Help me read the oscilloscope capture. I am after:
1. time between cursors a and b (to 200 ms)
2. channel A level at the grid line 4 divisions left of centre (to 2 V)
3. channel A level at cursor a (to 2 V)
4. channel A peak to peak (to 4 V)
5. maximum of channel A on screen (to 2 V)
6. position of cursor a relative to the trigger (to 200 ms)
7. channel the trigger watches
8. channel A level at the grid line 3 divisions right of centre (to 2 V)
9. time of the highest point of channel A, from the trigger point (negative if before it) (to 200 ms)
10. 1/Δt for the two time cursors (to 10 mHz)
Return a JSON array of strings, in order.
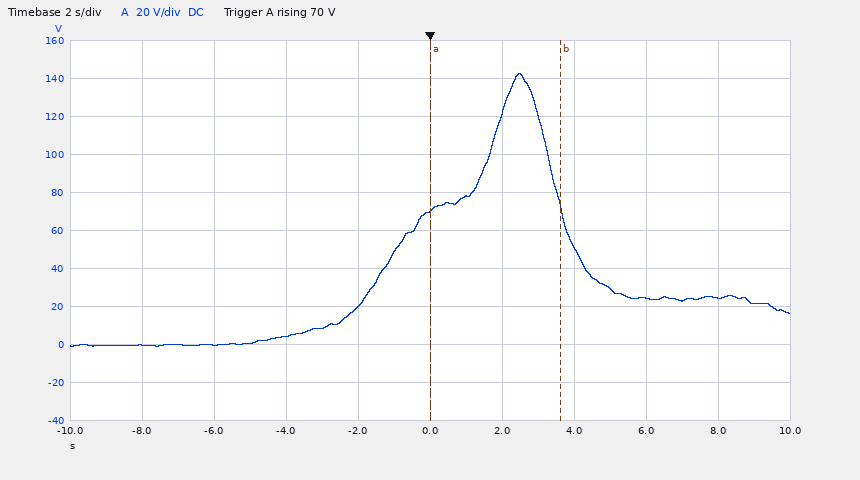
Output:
["3.6 s", "0 V", "70 V", "144 V", "142 V", "0.0 s", "channel A", "24 V", "+2.4 s", "280 mHz"]
